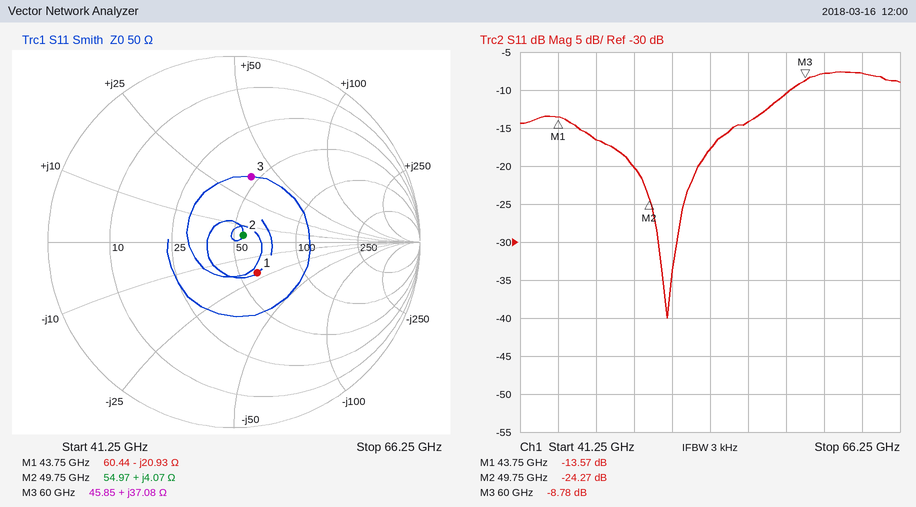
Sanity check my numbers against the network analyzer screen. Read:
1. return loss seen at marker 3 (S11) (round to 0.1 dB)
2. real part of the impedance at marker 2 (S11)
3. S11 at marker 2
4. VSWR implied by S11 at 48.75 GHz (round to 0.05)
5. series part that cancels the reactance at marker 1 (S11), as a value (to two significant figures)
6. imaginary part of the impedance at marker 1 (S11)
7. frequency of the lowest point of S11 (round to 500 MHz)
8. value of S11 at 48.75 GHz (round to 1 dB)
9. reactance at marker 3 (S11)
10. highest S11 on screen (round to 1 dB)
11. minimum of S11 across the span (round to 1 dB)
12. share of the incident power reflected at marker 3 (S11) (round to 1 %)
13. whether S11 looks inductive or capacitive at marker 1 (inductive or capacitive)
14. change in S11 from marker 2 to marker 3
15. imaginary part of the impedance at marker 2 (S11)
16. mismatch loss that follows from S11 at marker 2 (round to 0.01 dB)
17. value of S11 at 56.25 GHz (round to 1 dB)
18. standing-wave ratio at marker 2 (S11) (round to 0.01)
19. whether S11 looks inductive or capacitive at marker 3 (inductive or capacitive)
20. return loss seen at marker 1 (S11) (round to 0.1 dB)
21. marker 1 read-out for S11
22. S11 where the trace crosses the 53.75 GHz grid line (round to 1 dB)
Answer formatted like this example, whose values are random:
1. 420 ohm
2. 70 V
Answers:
1. 8.8 dB
2. 54.97 Ω
3. -24.27 dB
4. 1.20
5. 76 pH
6. -20.93 Ω
7. 51.0 GHz
8. -20 dB
9. +37.08 Ω
10. -8 dB
11. -40 dB
12. 13 %
13. capacitive
14. 15.49 dB
15. +4.07 Ω
16. 0.02 dB
17. -14 dB
18. 1.13
19. inductive
20. 13.6 dB
21. -13.57 dB
22. -18 dB
